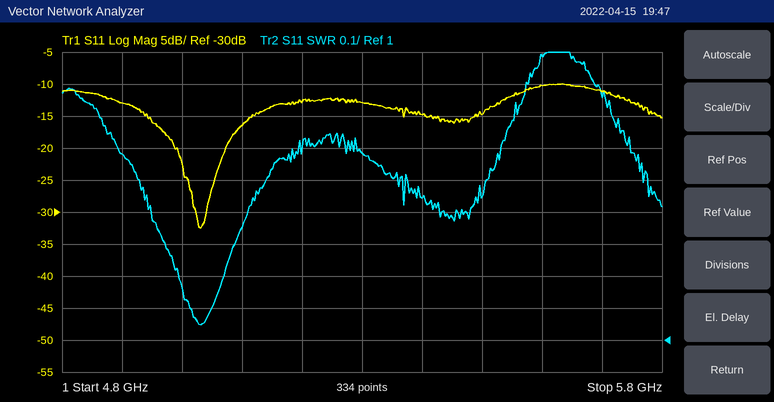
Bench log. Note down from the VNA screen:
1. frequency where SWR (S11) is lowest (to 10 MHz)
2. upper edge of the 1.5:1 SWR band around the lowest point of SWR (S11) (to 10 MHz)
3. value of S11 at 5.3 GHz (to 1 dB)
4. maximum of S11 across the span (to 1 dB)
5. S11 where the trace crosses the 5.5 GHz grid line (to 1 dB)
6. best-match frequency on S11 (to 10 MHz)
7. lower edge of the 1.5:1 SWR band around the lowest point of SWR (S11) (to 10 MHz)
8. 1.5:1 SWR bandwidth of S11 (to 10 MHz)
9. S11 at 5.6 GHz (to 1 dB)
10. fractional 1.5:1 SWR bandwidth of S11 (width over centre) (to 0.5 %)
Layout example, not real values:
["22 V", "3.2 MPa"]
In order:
["5.03 GHz", "5.14 GHz", "-13 dB", "-10 dB", "-15 dB", "5.03 GHz", "4.93 GHz", "210 MHz", "-10 dB", "4.0 %"]
